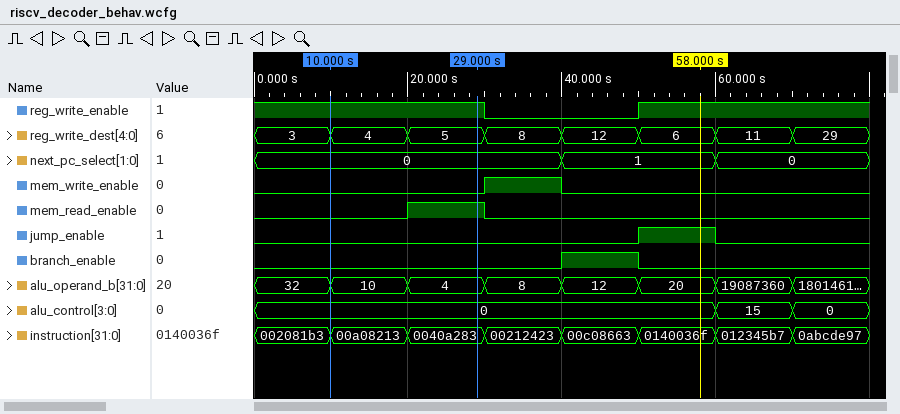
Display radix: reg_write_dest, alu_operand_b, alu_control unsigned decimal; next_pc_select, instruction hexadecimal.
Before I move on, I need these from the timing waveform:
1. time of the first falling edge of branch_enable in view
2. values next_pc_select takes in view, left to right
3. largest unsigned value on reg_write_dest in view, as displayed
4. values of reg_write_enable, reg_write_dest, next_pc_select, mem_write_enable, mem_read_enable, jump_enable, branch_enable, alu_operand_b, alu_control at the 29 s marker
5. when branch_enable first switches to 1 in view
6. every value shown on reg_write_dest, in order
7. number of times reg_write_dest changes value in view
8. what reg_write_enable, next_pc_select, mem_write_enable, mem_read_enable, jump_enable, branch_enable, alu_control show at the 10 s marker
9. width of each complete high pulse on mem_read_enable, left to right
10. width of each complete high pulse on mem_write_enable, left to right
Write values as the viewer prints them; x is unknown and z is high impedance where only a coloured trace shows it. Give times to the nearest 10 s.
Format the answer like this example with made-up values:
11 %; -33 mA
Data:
50 s; 0, 1, 0; 29; reg_write_enable=1, reg_write_dest=5, next_pc_select=0, mem_write_enable=0, mem_read_enable=1, jump_enable=0, branch_enable=0, alu_operand_b=4, alu_control=0; 40 s; 3, 4, 5, 8, 12, 6, 11, 29; 7; reg_write_enable=1, next_pc_select=0, mem_write_enable=0, mem_read_enable=0, jump_enable=0, branch_enable=0, alu_control=0; 10 s; 10 s
